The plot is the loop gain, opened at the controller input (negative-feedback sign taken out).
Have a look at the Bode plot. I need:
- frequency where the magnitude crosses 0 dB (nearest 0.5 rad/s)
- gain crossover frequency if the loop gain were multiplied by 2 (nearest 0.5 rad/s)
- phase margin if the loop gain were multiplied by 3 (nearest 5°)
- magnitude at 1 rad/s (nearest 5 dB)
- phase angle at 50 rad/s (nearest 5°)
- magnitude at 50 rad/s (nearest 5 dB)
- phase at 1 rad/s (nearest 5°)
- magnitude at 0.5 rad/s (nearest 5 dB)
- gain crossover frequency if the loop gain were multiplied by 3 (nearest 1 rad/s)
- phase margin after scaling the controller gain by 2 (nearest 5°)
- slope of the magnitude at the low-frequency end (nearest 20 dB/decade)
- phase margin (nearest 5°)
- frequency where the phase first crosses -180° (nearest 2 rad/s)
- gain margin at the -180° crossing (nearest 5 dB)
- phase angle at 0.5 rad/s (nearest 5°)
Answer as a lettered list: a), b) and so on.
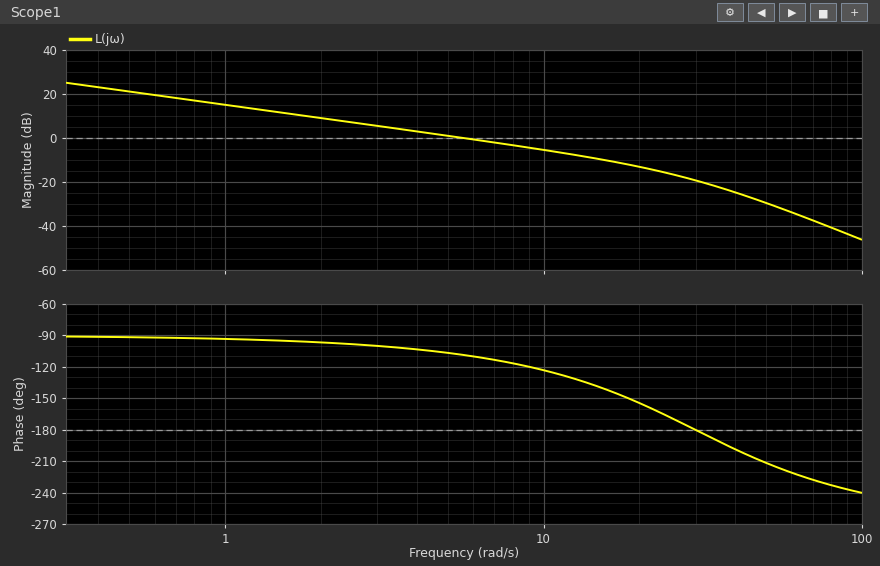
a) 5.5 rad/s
b) 10.5 rad/s
c) 40°
d) 15 dB
e) -210°
f) -30 dB
g) -95°
h) 20 dB
i) 15 rad/s
j) 55°
k) -20 dB/decade
l) 70°
m) 30 rad/s
n) 20 dB
o) -90°
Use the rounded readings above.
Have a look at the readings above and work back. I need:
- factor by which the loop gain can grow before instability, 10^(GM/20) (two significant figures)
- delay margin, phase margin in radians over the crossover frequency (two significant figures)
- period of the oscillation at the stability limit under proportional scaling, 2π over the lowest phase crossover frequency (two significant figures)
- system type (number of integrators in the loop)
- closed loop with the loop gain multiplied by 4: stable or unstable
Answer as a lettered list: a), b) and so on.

a) 10
b) 0.22 s
c) 0.21 s
d) 1
e) stable
